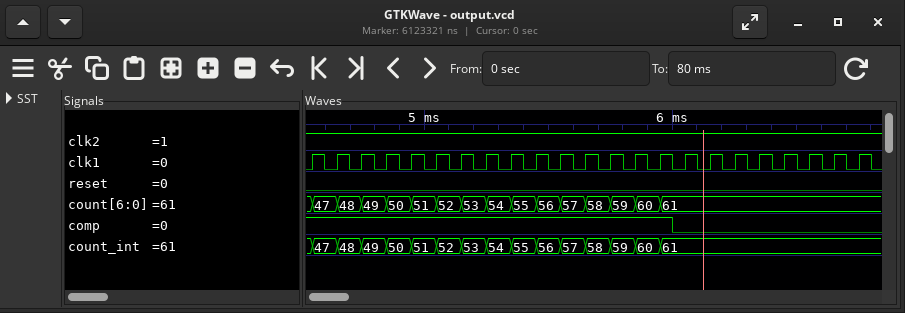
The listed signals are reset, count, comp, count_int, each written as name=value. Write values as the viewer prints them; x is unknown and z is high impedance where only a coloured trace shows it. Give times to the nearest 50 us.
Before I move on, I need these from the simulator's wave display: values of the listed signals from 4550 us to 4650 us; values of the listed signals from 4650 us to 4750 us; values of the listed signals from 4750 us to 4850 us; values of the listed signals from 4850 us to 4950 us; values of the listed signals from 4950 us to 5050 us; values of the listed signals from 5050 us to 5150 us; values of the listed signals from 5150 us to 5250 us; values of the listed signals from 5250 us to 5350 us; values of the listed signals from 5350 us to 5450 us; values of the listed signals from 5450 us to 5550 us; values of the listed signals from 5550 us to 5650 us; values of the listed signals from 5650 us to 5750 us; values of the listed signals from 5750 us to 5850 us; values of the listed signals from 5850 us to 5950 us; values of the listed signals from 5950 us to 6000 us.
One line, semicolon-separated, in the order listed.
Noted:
reset=0, count=47, comp=1, count_int=47; reset=0, count=48, comp=1, count_int=48; reset=0, count=49, comp=1, count_int=49; reset=0, count=50, comp=1, count_int=50; reset=0, count=51, comp=1, count_int=51; reset=0, count=52, comp=1, count_int=52; reset=0, count=53, comp=1, count_int=53; reset=0, count=54, comp=1, count_int=54; reset=0, count=55, comp=1, count_int=55; reset=0, count=56, comp=1, count_int=56; reset=0, count=57, comp=1, count_int=57; reset=0, count=58, comp=1, count_int=58; reset=0, count=59, comp=1, count_int=59; reset=0, count=60, comp=1, count_int=60; reset=0, count=61, comp=1, count_int=61
